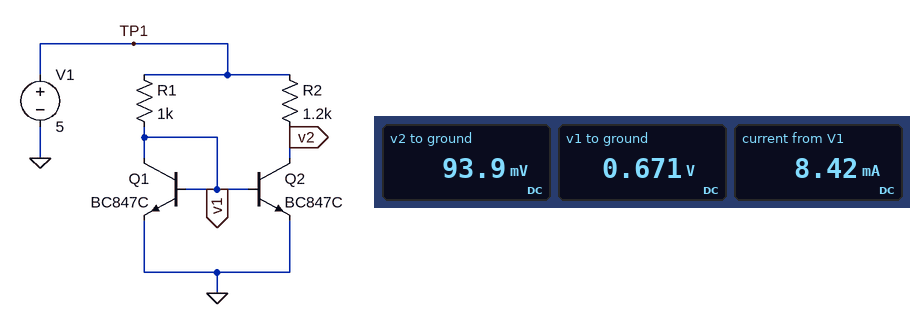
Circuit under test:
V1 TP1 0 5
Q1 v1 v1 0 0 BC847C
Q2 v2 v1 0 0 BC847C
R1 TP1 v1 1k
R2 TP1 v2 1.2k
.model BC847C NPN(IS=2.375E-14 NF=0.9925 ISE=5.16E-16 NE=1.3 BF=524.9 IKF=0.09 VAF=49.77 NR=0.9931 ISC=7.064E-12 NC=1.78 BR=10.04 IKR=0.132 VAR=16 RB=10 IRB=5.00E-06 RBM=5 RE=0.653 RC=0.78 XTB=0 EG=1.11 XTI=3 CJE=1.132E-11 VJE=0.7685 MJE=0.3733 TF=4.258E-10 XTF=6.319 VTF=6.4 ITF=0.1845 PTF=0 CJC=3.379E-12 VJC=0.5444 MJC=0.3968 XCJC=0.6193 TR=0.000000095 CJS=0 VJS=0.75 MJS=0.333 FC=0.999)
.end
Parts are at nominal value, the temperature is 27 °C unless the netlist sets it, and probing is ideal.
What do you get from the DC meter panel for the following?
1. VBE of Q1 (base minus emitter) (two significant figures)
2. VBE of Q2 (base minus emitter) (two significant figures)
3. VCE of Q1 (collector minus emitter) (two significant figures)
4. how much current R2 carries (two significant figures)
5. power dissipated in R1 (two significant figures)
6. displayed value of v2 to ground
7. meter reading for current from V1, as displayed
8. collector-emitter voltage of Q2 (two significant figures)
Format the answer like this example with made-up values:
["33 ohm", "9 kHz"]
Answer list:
["670 mV", "670 mV", "670 mV", "4.1 mA", "19 mW", "93.9 mV", "8.42 mA", "94 mV"]
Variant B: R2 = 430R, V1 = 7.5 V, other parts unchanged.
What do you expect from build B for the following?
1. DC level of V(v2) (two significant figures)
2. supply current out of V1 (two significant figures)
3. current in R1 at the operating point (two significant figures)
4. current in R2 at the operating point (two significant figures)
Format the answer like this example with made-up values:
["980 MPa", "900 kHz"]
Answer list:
["4.4 V", "14 mA", "6.8 mA", "7.2 mA"]
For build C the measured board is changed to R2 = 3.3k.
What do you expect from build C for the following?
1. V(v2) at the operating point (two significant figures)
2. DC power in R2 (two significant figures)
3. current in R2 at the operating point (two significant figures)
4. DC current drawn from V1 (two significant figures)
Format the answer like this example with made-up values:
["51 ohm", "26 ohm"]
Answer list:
["17 mV", "7.5 mW", "1.5 mA", "5.8 mA"]
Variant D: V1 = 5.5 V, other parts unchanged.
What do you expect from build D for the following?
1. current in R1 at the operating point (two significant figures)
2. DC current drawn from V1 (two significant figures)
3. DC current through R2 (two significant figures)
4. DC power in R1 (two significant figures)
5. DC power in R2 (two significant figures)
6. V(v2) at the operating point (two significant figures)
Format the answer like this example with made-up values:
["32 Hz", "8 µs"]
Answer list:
["4.8 mA", "9.3 mA", "4.5 mA", "23 mW", "24 mW", "89 mV"]
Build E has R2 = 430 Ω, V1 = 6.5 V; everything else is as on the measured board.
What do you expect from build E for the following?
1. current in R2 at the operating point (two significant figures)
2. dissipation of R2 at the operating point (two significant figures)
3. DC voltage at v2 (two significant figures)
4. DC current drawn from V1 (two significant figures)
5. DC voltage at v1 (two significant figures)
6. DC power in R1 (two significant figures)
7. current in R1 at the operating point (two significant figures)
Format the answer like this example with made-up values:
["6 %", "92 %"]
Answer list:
["6.1 mA", "16 mW", "3.9 V", "12 mA", "680 mV", "34 mW", "5.8 mA"]
